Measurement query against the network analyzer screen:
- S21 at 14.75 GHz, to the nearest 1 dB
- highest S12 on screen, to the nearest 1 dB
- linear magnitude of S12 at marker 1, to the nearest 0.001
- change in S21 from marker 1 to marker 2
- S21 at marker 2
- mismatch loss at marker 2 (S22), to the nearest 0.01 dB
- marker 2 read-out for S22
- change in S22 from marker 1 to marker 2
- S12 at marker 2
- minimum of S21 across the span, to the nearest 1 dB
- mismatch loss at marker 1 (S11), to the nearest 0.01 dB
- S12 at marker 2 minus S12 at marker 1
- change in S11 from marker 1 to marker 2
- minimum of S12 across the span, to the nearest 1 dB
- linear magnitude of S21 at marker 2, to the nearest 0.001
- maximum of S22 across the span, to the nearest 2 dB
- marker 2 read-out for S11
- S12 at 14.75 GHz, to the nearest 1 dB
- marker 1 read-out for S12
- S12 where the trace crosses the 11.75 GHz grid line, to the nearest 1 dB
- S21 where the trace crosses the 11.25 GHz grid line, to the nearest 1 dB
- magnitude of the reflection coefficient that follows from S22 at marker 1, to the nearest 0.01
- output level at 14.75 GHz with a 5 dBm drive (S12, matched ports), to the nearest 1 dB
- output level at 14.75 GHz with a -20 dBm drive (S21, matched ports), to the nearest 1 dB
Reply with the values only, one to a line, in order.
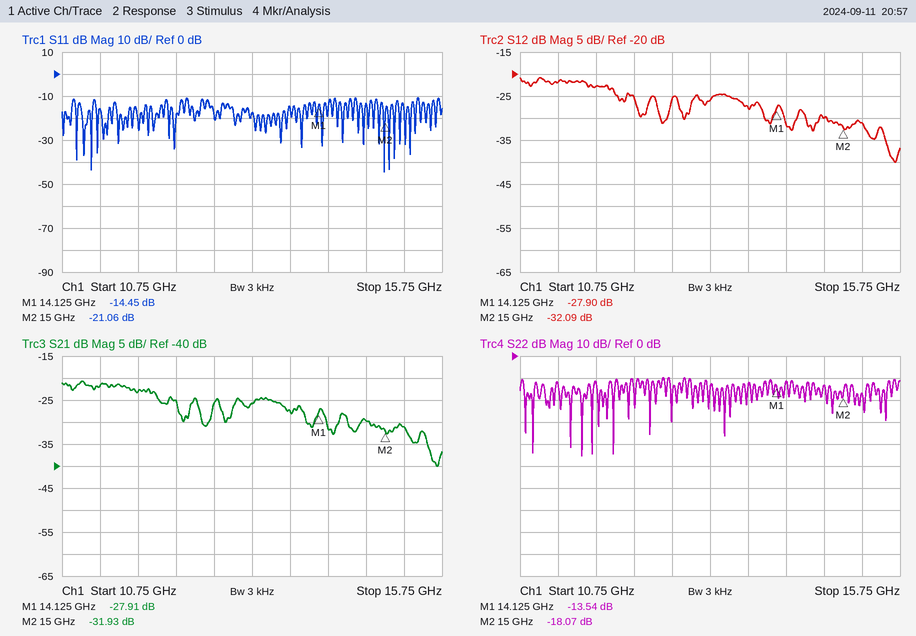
-30 dB
-21 dB
0.040
-4.02 dB
-31.93 dB
0.07 dB
-18.07 dB
-4.53 dB
-32.09 dB
-40 dB
0.16 dB
-4.19 dB
-6.61 dB
-40 dB
0.025
-10 dB
-21.06 dB
-30 dB
-27.90 dB
-23 dB
-22 dB
0.21
-25 dBm
-50 dBm
